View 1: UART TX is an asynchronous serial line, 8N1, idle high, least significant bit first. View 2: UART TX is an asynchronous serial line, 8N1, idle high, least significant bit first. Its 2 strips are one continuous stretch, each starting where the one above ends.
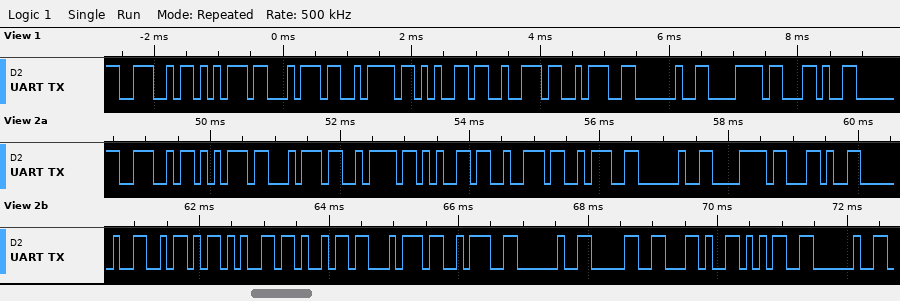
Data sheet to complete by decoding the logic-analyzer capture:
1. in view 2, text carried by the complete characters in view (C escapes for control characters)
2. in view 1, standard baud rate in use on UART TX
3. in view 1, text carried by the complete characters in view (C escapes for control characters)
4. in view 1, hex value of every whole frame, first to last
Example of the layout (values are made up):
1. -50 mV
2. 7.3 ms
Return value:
1. "Nutzer: x, Zeit: 0,5 "
2. 9600 baud
3. "Nutzer: x,"
4. 0x4E 0x75 0x74 0x7A 0x65 0x72 0x3A 0x20 0x78 0x2C
